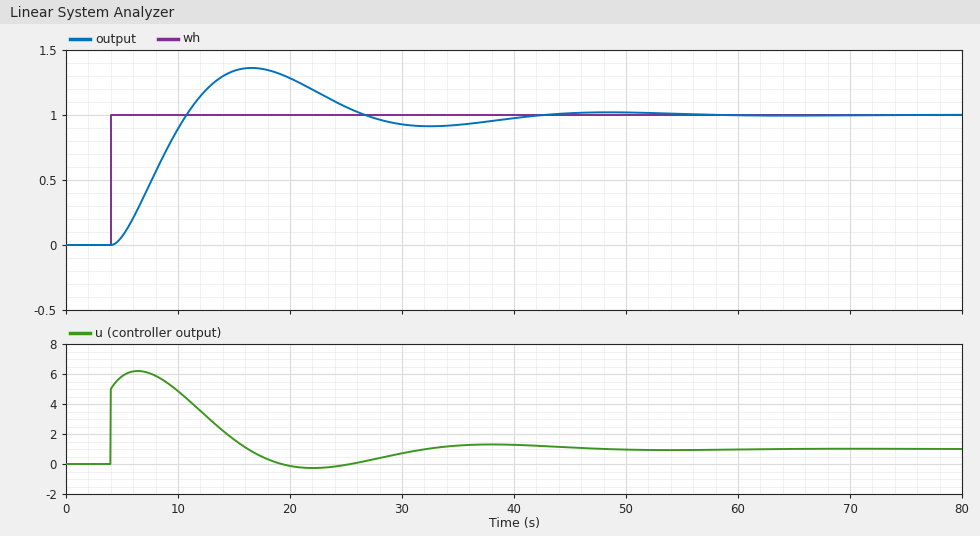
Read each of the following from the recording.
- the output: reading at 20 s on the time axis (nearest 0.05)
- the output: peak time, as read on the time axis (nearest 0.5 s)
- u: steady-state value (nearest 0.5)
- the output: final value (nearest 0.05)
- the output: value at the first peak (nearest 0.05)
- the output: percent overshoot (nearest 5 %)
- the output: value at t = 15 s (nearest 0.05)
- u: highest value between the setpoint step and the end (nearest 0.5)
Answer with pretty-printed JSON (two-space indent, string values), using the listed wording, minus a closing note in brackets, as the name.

{
  "the output: reading at 20 s on the time axis": "1.30",
  "the output: peak time, as read on the time axis": "16.5 s",
  "u: steady-state value": "1.0",
  "the output: final value": "1.00",
  "the output: value at the first peak": "1.35",
  "the output: percent overshoot": "35 %",
  "the output: value at t = 15 s": "1.35",
  "u: highest value between the setpoint step and the end": "6.0"
}
